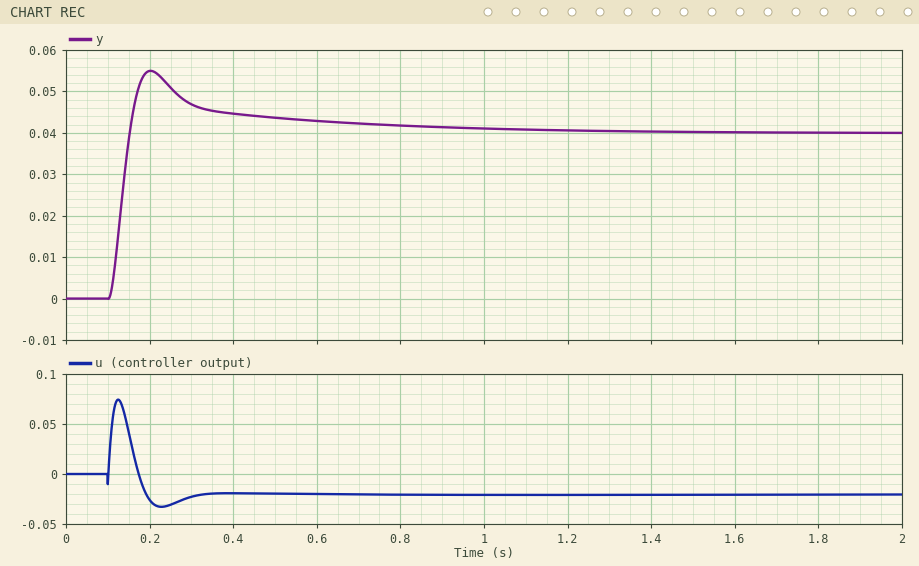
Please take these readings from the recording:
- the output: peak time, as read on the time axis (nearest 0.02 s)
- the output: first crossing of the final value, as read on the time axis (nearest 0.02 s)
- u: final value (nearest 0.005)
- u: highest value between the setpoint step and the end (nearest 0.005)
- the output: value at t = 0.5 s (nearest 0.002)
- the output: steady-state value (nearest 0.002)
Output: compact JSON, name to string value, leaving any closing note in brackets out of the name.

{"the output: peak time, as read on the time axis": "0.20 s", "the output: first crossing of the final value, as read on the time axis": "0.16 s", "u: final value": "-0.020", "u: highest value between the setpoint step and the end": "0.075", "the output: value at t = 0.5 s": "0.044", "the output: steady-state value": "0.040"}
